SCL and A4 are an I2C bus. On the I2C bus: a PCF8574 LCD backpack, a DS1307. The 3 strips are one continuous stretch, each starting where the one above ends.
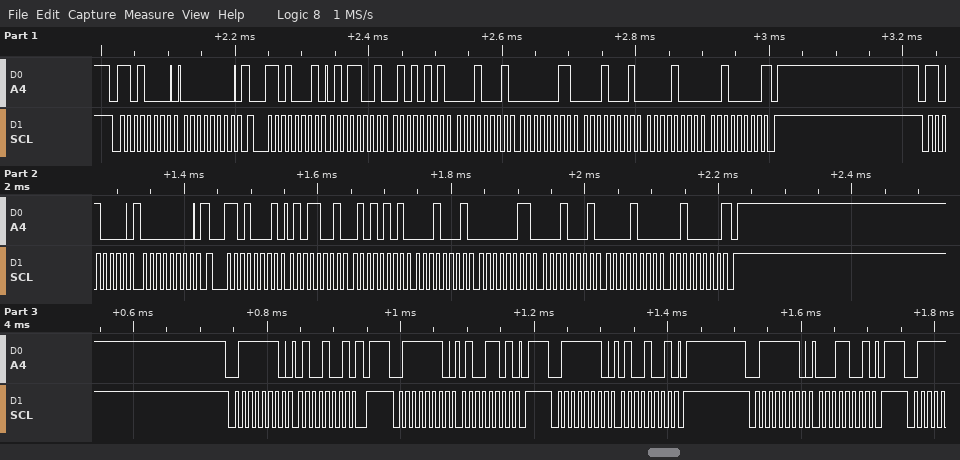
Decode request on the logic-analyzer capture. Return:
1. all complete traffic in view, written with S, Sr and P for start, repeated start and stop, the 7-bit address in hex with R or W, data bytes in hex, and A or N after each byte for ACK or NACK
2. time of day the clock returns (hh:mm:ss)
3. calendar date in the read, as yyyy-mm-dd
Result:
S 68W A 00 A Sr 68R A 59 A 55 A 11 A 03 A 11 A 08 A 20 N P S 68W A 00 A Sr 68R A 59 A 55 A 11 A 03 A 11 A 08 A 20 N P S 3FW A 49 A P S 3FW A 4D A P S 3FW A 49 A P S 3FW A 19 A P
11:55:59
2020-08-11
